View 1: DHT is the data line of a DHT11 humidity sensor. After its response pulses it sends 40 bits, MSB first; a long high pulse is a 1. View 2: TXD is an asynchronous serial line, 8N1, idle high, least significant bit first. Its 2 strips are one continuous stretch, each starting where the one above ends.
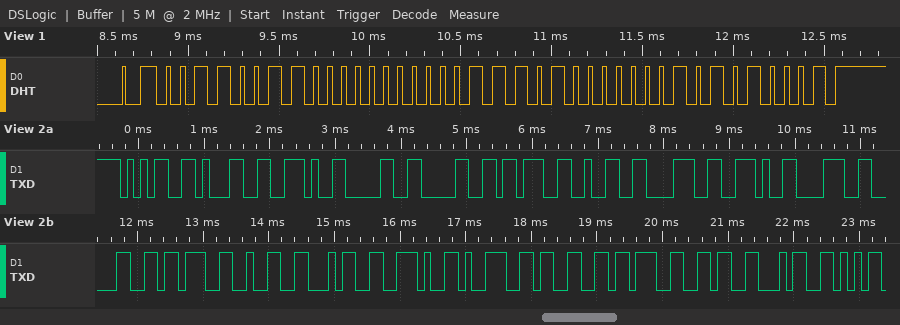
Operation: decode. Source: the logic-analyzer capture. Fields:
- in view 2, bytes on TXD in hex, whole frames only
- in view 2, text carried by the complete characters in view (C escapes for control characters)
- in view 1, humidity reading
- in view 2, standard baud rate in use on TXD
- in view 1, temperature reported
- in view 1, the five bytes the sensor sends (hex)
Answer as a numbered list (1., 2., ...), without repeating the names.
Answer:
1. 35 31 2E 30 30 3B 32 38 2E 38 30 3B 32 34 2E 39 33 3B 36 34
2. "51.00;28.80;24.93;64"
3. 51 %
4. 9600 baud
5. 29.1 °C
6. 33 00 1D 01 51
